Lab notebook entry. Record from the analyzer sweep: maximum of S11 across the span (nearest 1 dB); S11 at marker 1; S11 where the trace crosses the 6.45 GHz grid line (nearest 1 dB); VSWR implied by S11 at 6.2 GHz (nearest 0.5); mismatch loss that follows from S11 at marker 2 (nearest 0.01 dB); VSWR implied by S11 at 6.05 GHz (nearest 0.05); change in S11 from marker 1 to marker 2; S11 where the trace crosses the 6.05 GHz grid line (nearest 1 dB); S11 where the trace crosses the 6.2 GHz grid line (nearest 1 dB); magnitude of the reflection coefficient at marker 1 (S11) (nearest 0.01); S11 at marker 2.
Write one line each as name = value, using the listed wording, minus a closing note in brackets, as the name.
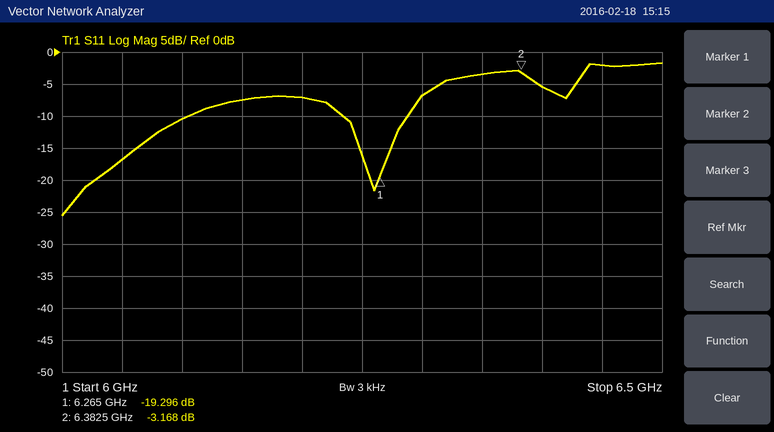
maximum of S11 across the span = -2 dB
S11 at marker 1 = -19.296 dB
S11 where the trace crosses the 6.45 GHz grid line = -2 dB
VSWR implied by S11 at 6.2 GHz = 2.5
mismatch loss that follows from S11 at marker 2 = 2.86 dB
VSWR implied by S11 at 6.05 GHz = 1.35
change in S11 from marker 1 to marker 2 = 16.128 dB
S11 where the trace crosses the 6.05 GHz grid line = -17 dB
S11 where the trace crosses the 6.2 GHz grid line = -7 dB
magnitude of the reflection coefficient at marker 1 (S11) = 0.11
S11 at marker 2 = -3.168 dB
